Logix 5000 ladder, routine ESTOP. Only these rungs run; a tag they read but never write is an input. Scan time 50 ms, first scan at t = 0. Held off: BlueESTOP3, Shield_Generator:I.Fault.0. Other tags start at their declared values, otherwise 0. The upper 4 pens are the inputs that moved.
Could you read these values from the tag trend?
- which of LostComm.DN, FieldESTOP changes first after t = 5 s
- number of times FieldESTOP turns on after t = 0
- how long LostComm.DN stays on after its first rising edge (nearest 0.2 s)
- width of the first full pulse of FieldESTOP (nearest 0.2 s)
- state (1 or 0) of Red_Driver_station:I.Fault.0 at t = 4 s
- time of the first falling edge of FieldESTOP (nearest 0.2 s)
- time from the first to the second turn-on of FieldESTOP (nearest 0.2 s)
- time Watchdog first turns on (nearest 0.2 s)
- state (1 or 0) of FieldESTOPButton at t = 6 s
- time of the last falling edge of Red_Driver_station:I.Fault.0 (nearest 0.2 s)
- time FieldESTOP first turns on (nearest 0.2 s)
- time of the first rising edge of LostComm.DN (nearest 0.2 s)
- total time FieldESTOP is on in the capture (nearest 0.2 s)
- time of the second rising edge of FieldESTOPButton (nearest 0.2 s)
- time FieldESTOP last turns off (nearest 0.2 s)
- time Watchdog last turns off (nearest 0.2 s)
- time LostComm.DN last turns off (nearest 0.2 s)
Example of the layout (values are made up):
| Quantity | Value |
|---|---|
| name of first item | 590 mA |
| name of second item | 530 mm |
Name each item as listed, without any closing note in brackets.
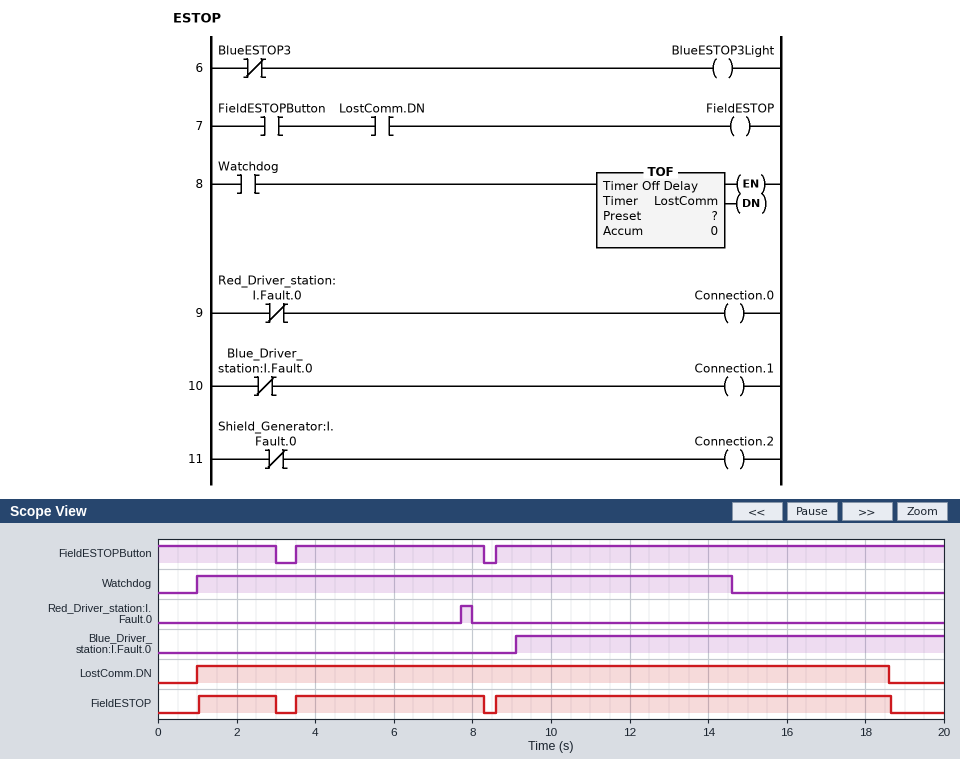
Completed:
| Quantity | Value |
|---|---|
| which of LostComm.DN, FieldESTOP changes first after t = 5 s | FieldESTOP |
| number of times FieldESTOP turns on after t = 0 | 3 |
| how long LostComm.DN stays on after its first rising edge | 17.6 s |
| width of the first full pulse of FieldESTOP | 2.0 s |
| state (1 or 0) of Red_Driver_station:I.Fault.0 at t = 4 s | 0 |
| time of the first falling edge of FieldESTOP | 3.0 s |
| time from the first to the second turn-on of FieldESTOP | 2.4 s |
| time Watchdog first turns on | 1.0 s |
| state (1 or 0) of FieldESTOPButton at t = 6 s | 1 |
| time of the last falling edge of Red_Driver_station:I.Fault.0 | 8.0 s |
| time FieldESTOP first turns on | 1.0 s |
| time of the first rising edge of LostComm.DN | 1.0 s |
| total time FieldESTOP is on in the capture | 16.8 s |
| time of the second rising edge of FieldESTOPButton | 8.6 s |
| time FieldESTOP last turns off | 18.6 s |
| time Watchdog last turns off | 14.6 s |
| time LostComm.DN last turns off | 18.6 s |
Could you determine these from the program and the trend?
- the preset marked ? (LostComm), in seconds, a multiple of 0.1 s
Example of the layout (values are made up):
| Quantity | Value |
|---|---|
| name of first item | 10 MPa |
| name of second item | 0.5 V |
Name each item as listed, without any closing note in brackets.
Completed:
| Quantity | Value |
|---|---|
| the preset marked ? (LostComm), in seconds, a multiple of 0.1 s | 4.0 s |
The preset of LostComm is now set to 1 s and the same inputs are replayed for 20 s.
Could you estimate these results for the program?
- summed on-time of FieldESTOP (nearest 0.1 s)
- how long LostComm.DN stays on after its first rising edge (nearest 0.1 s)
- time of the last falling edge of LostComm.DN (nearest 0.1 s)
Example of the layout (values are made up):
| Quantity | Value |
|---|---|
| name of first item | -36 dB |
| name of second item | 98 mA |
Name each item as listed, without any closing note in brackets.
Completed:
| Quantity | Value |
|---|---|
| summed on-time of FieldESTOP | 13.8 s |
| how long LostComm.DN stays on after its first rising edge | 14.6 s |
| time of the last falling edge of LostComm.DN | 15.6 s |
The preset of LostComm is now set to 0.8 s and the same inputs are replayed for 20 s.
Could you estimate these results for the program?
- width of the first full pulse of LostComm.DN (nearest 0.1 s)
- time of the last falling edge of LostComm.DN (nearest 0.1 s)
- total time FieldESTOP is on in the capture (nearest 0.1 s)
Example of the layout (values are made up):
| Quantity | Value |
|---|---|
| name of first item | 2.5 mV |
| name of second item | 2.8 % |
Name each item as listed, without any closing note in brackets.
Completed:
| Quantity | Value |
|---|---|
| width of the first full pulse of LostComm.DN | 14.4 s |
| time of the last falling edge of LostComm.DN | 15.4 s |
| total time FieldESTOP is on in the capture | 13.6 s |
